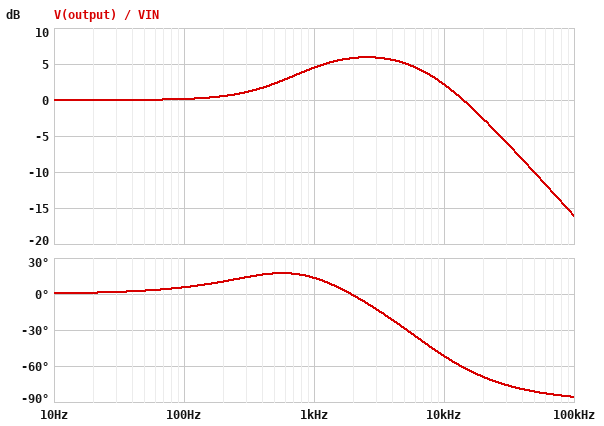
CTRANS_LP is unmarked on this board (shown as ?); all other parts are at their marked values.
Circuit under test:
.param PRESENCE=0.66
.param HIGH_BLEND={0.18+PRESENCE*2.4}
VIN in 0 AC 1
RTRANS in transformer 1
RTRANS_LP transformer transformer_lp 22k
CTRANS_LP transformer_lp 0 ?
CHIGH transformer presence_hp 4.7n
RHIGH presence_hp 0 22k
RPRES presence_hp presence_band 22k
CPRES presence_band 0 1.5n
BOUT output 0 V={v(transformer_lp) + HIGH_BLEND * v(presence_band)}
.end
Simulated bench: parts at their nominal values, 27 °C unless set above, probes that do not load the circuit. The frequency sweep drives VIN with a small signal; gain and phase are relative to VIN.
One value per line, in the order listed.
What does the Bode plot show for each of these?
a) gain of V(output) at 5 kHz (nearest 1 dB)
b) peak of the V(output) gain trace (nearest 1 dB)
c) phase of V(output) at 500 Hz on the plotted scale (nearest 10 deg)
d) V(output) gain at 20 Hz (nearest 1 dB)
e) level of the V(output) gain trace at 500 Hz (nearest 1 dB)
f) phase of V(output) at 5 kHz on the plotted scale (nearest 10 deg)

5 dB
6 dB
20 deg
0 dB
2 dB
-30 deg
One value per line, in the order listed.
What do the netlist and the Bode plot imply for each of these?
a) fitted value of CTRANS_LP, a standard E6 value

1 nF
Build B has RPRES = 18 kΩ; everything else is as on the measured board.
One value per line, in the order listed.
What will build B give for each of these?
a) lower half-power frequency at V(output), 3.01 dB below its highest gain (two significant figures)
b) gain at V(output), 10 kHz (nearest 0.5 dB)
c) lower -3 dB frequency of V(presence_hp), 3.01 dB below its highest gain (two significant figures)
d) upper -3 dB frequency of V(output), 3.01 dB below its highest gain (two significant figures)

640 Hz
3.0 dB
2.9 kHz
9.6 kHz
